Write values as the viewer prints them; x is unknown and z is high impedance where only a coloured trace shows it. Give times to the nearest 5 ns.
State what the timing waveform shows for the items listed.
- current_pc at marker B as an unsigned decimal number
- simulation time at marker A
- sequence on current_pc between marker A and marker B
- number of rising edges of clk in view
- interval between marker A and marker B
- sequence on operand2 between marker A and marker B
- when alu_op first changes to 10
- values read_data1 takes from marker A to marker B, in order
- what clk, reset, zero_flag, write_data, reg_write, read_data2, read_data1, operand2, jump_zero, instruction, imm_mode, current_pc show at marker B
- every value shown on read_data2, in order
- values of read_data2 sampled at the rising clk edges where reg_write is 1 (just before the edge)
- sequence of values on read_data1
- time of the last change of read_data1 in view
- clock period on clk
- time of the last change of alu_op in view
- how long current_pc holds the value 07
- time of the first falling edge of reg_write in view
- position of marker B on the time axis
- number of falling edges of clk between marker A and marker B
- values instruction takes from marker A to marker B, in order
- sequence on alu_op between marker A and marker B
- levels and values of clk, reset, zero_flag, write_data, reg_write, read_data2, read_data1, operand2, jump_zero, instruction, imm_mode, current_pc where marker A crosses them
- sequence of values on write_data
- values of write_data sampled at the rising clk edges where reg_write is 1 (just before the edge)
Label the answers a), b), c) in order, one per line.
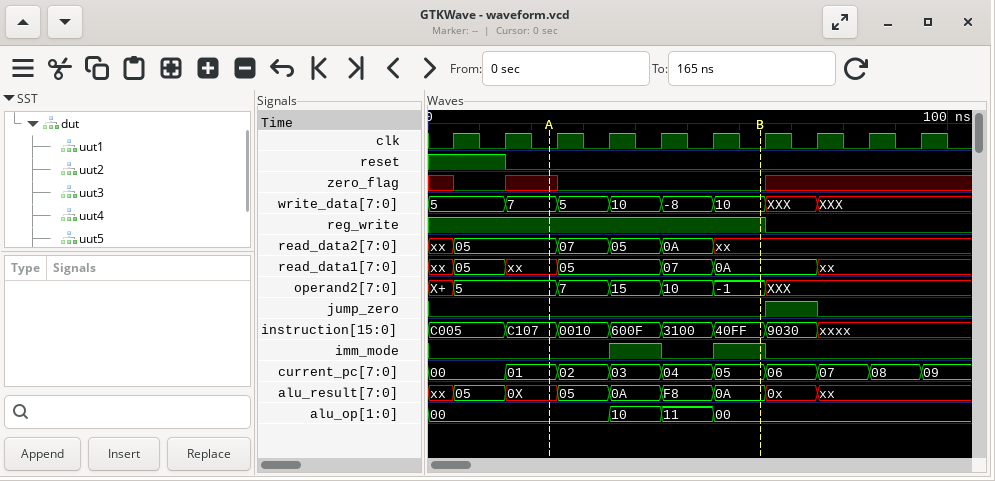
a) 5
b) 25 ns
c) 01, 02, 03, 04, 05
d) 10
e) 40 ns
f) 5, 7, 15, 10, -1
g) 35 ns
h) xx, 05, 07, 0A
i) clk=0, reset=0, zero_flag=0, write_data=10, reg_write=1, read_data2=xx, read_data1=0A, operand2=-1, jump_zero=0, instruction=40FF, imm_mode=1, current_pc=05
j) xx, 05, 07, 05, 0A, xx
k) xx, 05, 05, 07, 05, 0A, xx
l) xx, 05, xx, 05, 07, 0A, xx
m) 75 ns
n) 10 ns
o) 55 ns
p) 10 ns
q) 65 ns
r) 65 ns
s) 4
t) C107, 0010, 600F, 3100, 40FF
u) 00, 10, 11, 00
v) clk=0, reset=0, zero_flag=x, write_data=7, reg_write=1, read_data2=05, read_data1=xx, operand2=5, jump_zero=0, instruction=C107, imm_mode=0, current_pc=01
w) 5, 7, 5, 10, -8, 10, XXX, XXX
x) 5, 5, 7, 5, 10, -8, 10
